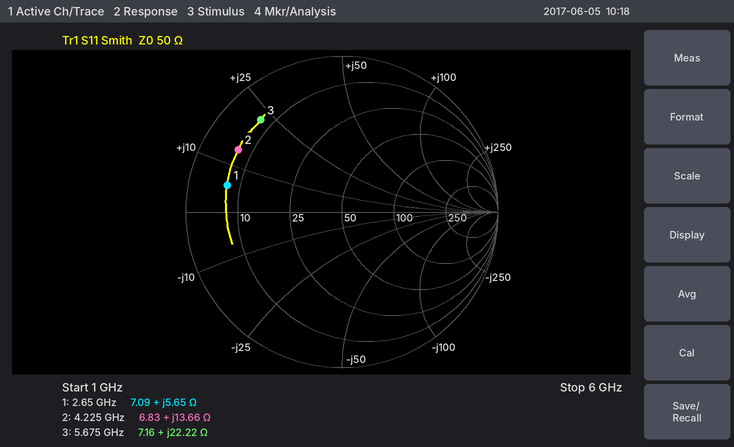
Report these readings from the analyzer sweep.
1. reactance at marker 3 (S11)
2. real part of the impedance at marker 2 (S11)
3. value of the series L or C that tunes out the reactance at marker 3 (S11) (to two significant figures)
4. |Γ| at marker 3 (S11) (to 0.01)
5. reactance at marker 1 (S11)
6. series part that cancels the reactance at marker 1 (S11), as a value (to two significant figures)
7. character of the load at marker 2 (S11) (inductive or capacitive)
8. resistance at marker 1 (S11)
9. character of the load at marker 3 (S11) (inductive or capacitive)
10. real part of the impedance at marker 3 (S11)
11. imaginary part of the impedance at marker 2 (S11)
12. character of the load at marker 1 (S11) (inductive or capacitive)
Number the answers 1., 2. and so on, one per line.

1. +22.22 Ω
2. 6.83 Ω
3. 1.3 pF
4. 0.79
5. +5.65 Ω
6. 11 pF
7. inductive
8. 7.09 Ω
9. inductive
10. 7.16 Ω
11. +13.66 Ω
12. inductive
